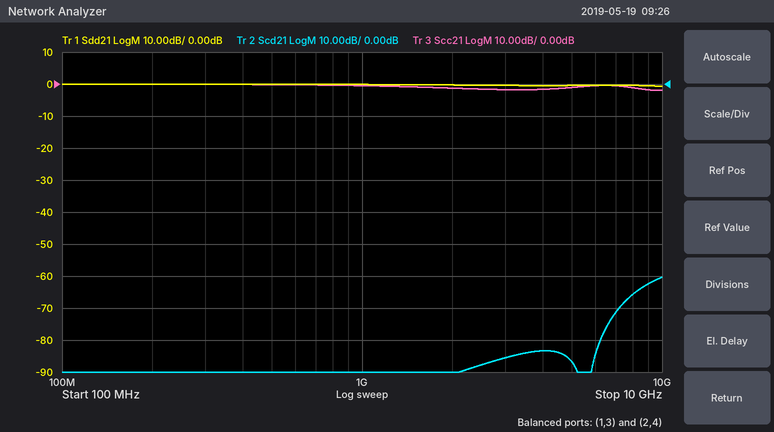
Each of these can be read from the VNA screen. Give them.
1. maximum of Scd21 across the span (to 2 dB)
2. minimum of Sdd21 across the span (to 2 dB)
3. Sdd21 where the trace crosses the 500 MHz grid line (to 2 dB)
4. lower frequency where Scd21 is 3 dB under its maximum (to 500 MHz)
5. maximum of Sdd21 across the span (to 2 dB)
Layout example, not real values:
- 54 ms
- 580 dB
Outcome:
- -60 dB
- 0 dB
- 0 dB
- 8.5 GHz
- 0 dB
